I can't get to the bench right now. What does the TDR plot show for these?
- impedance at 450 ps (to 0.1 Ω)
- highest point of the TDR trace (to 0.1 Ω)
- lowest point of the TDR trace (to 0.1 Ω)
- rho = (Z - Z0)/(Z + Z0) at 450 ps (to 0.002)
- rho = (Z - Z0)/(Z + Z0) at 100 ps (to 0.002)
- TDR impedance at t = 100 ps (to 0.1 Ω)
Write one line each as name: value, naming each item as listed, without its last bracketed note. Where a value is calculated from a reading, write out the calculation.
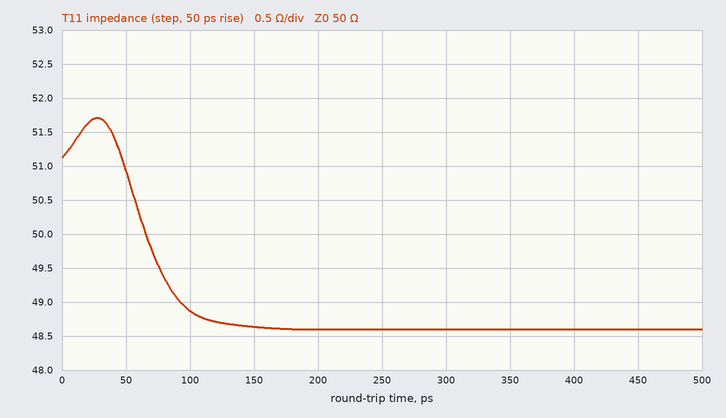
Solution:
impedance at 450 ps: 48.6 Ω
highest point of the TDR trace: 51.7 Ω
lowest point of the TDR trace: 48.6 Ω
rho = (Z - Z0)/(Z + Z0) at 450 ps: (48.6 − 50)/(48.6 + 50) ≈ -0.014
rho = (Z - Z0)/(Z + Z0) at 100 ps: (48.9 − 50)/(48.9 + 50) ≈ -0.0111, so -0.012 to the nearest 0.002
TDR impedance at t = 100 ps: 48.9 Ω
